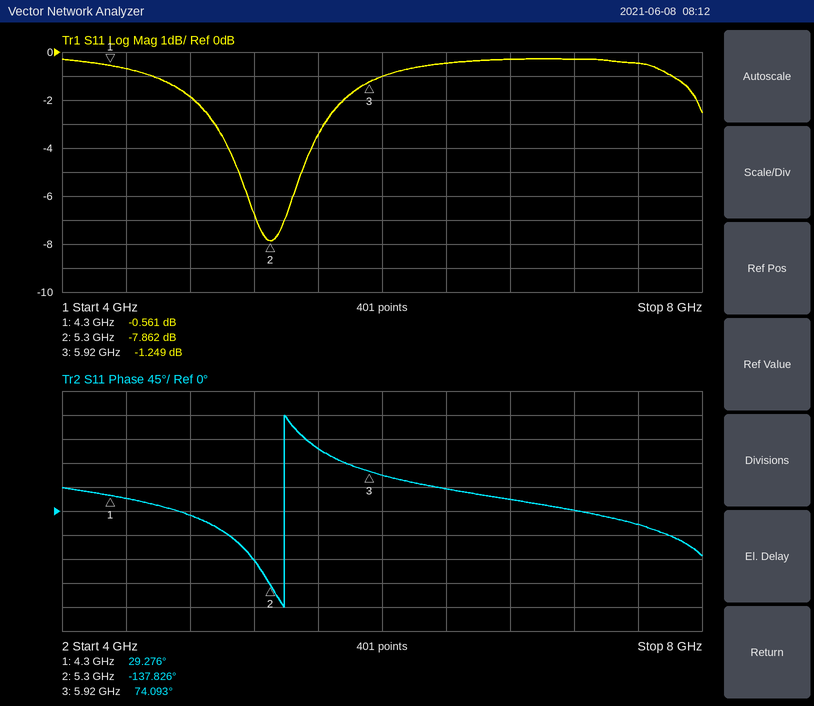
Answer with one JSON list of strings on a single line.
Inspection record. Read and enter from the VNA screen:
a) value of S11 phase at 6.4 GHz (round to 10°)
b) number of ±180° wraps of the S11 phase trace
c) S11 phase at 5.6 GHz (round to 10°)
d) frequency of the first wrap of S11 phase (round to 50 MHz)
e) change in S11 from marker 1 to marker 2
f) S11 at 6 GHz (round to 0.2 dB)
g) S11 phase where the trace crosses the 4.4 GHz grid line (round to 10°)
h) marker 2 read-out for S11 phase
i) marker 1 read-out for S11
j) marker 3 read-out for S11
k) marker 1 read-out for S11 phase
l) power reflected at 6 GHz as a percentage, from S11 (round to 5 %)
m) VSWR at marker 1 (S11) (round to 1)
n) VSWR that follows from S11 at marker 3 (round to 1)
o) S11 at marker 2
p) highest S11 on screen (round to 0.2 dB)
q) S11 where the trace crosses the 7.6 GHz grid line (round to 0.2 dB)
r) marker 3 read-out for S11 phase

["40°", "1", "120°", "5.40 GHz", "-7.301 dB", "-1.0 dB", "20°", "-137.826°", "-0.561 dB", "-1.249 dB", "29.276°", "80 %", "31", "14", "-7.862 dB", "-0.2 dB", "-0.4 dB", "74.093°"]
